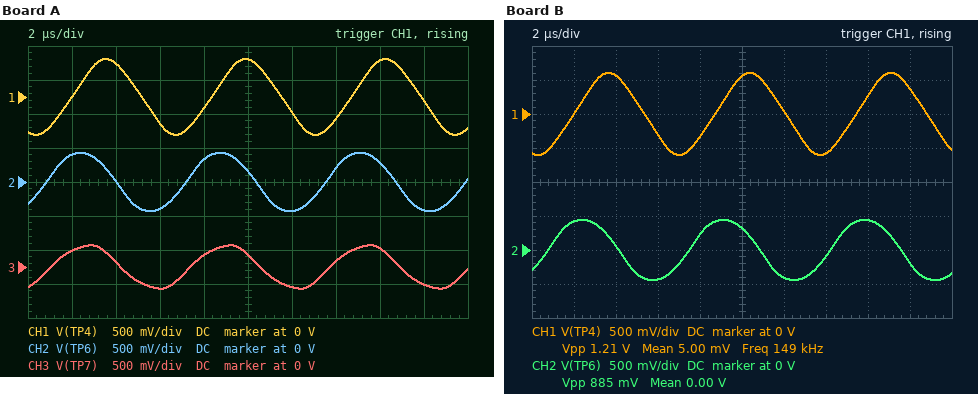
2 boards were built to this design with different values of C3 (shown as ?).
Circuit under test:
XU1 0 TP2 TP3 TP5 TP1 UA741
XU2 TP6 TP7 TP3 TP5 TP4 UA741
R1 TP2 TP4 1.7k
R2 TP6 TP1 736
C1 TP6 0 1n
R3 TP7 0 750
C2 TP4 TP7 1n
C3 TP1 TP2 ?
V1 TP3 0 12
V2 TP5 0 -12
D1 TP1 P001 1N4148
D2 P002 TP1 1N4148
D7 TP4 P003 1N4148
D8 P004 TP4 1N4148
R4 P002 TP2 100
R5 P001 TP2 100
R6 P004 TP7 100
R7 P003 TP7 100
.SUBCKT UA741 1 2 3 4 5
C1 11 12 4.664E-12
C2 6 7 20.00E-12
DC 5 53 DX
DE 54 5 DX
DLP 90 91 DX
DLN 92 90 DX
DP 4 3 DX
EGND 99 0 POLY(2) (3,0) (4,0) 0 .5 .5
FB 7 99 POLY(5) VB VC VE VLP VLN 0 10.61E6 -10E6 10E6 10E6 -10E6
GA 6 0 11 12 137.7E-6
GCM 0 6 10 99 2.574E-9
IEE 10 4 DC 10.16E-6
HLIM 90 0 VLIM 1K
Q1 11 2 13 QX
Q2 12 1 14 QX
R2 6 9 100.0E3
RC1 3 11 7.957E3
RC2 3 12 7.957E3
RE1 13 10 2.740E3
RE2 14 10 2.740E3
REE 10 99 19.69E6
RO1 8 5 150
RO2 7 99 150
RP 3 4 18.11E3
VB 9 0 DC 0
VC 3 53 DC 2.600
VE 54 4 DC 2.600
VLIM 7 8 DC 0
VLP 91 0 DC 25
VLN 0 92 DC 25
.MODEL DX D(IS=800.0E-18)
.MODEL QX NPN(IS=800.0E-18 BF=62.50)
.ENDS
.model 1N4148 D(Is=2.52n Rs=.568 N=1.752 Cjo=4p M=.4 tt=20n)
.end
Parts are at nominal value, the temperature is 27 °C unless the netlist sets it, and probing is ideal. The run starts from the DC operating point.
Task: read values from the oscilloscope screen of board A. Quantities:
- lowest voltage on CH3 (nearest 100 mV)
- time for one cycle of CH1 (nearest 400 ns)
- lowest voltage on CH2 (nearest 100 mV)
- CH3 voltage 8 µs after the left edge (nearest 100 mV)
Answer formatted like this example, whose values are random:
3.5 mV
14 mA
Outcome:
-300 mV
6.4 µs
-400 mV
200 mV
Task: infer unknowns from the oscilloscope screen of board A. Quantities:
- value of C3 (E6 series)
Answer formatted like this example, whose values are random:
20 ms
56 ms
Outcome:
220 pF
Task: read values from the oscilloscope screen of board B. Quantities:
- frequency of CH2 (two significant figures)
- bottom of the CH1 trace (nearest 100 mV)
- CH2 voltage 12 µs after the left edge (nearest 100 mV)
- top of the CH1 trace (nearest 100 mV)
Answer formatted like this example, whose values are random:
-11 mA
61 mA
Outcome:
150 kHz
-600 mV
-400 mV
600 mV
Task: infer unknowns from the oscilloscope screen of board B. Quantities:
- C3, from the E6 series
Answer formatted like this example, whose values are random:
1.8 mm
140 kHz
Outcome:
330 pF
